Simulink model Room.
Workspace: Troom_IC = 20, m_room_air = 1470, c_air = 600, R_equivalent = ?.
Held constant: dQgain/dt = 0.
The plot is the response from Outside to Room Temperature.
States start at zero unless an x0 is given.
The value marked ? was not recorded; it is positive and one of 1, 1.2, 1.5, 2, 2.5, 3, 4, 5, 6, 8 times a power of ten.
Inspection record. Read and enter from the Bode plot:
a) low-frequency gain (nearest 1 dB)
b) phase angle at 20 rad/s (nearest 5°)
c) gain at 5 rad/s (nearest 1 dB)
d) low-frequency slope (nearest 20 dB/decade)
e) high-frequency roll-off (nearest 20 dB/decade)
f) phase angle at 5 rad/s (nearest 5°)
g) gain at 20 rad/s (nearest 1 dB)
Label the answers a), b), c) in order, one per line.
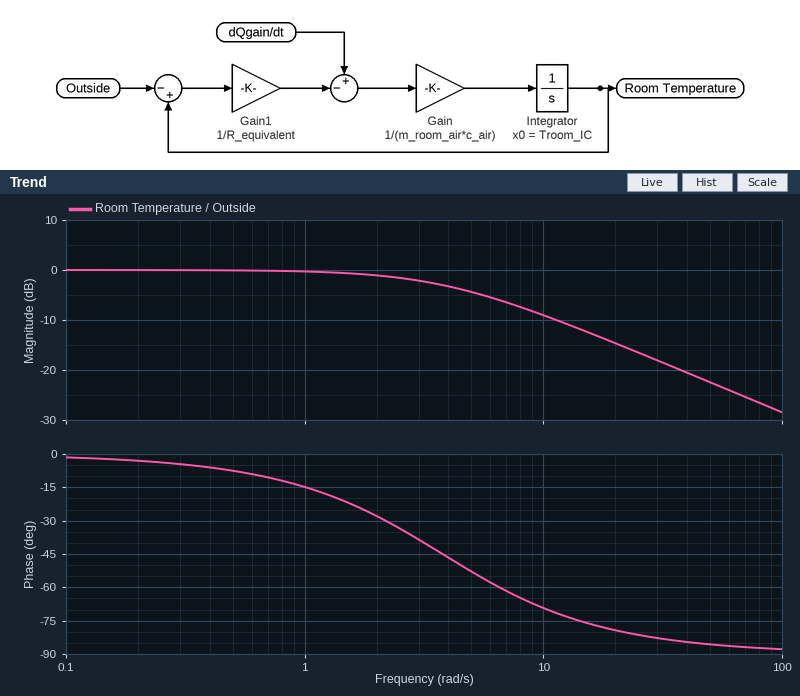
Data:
a) 0 dB
b) -80°
c) -4 dB
d) 0 dB/decade
e) -20 dB/decade
f) -55°
g) -15 dB
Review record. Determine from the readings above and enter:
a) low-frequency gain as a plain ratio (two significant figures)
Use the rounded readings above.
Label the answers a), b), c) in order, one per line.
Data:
a) 1.0
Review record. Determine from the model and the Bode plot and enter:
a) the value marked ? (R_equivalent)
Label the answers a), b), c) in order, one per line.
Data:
a) 3e-07
